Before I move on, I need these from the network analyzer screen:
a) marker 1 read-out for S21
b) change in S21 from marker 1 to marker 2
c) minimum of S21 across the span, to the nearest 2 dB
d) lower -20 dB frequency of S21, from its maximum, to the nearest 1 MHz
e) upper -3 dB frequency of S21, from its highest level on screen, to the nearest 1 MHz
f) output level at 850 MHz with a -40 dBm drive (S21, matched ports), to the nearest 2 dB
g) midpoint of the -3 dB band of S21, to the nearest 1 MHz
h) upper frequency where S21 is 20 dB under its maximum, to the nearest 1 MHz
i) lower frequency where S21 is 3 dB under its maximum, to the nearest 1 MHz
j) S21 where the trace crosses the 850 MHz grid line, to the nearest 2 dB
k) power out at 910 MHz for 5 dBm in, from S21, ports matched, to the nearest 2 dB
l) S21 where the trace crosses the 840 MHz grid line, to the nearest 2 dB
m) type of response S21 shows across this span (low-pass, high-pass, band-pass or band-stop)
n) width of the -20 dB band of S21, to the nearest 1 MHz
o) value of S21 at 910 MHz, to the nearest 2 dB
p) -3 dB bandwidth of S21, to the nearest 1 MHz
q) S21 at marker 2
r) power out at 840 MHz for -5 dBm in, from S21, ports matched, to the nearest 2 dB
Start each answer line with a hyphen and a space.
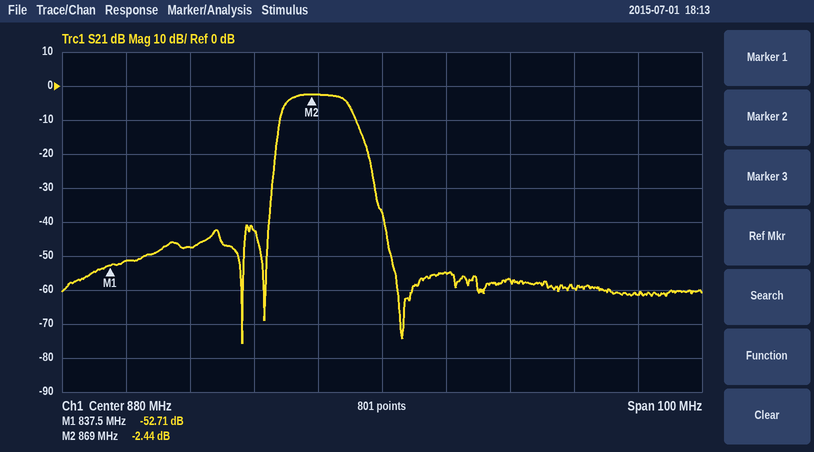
- -52.71 dB
- 50.27 dB
- -76 dB
- 863 MHz
- 875 MHz
- -88 dBm
- 870 MHz
- 878 MHz
- 865 MHz
- -48 dB
- -54 dBm
- -52 dB
- band-pass
- 15 MHz
- -60 dB
- 10 MHz
- -2.44 dB
- -56 dBm
